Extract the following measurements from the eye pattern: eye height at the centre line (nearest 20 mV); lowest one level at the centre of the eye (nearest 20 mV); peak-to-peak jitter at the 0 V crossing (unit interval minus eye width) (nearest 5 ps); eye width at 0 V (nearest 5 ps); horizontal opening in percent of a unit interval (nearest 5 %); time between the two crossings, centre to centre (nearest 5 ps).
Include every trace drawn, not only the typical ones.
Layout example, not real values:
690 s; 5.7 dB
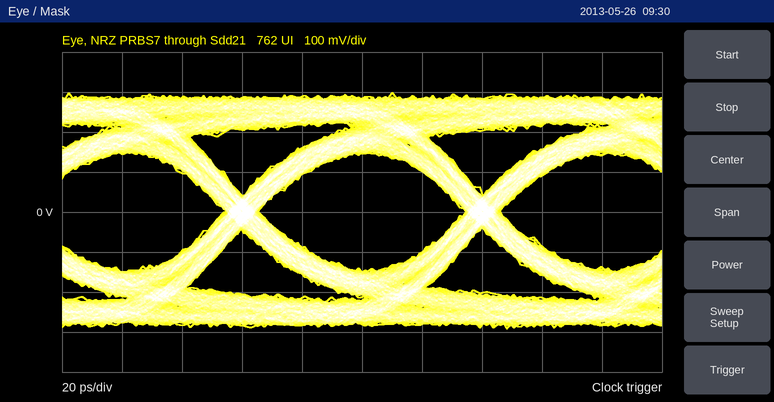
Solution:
300 mV; 140 mV; 10 ps; 70 ps; 85 %; 80 ps
